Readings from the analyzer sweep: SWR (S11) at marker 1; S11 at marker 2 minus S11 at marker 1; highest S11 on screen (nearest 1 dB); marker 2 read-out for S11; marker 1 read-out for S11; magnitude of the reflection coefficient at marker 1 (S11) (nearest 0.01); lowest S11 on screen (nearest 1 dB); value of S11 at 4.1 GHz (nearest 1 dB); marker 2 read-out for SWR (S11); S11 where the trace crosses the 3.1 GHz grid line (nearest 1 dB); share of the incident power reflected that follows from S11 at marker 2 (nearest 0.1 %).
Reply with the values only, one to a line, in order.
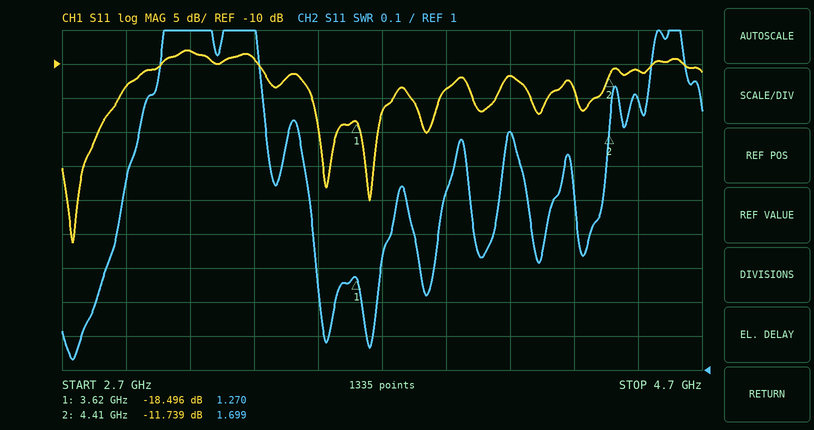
1.270
6.757 dB
-8 dB
-11.739 dB
-18.496 dB
0.12
-36 dB
-12 dB
1.699
-8 dB
6.7 %
